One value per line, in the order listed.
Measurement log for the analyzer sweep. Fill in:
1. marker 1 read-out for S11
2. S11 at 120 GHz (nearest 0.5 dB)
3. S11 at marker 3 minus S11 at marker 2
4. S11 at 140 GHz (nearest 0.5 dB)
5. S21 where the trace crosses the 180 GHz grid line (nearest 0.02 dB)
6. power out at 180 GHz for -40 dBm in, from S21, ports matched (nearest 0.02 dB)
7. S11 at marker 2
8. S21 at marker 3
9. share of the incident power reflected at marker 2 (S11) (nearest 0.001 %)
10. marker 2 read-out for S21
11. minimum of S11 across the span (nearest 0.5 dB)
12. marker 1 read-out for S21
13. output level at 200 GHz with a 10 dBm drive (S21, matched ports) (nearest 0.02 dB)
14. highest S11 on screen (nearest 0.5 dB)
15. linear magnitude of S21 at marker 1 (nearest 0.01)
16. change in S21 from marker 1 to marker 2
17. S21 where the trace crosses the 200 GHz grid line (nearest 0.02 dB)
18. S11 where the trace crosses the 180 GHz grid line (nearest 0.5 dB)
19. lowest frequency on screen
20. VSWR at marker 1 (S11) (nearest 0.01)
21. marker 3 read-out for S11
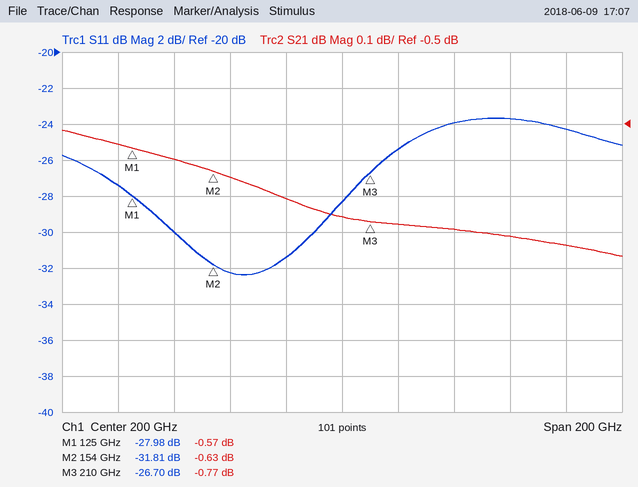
-27.98 dB
-27.5 dB
5.11 dB
-30.0 dB
-0.70 dB
-40.70 dBm
-31.81 dB
-0.77 dB
0.066 %
-0.63 dB
-32.5 dB
-0.57 dB
9.24 dBm
-23.5 dB
0.94
-0.06 dB
-0.76 dB
-31.5 dB
100 GHz
1.08
-26.70 dB
